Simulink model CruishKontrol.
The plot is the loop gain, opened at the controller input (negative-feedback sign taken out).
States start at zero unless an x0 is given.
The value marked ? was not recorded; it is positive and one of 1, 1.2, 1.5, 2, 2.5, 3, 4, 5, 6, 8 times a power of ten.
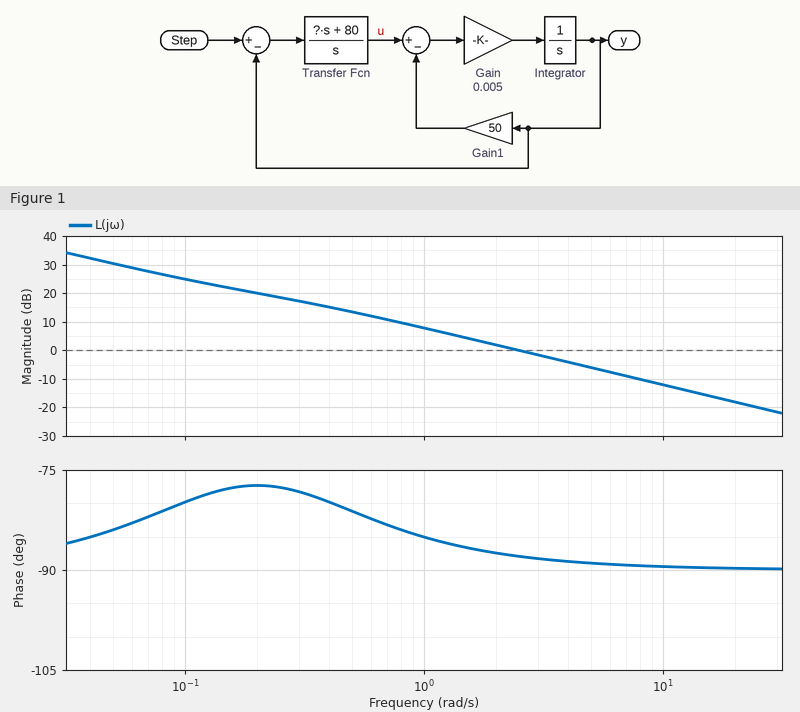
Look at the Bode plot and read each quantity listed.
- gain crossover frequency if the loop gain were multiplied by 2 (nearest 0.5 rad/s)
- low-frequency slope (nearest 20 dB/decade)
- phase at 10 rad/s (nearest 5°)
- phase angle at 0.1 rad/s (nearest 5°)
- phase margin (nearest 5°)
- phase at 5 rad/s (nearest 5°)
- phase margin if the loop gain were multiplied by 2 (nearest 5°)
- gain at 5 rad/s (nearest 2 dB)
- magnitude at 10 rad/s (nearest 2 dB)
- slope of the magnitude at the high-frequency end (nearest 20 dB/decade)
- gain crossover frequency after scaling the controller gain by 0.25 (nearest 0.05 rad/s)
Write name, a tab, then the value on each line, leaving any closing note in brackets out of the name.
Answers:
gain crossover frequency if the loop gain were multiplied by 2	5.0 rad/s
low-frequency slope	-20 dB/decade
phase at 10 rad/s	-90°
phase angle at 0.1 rad/s	-80°
phase margin	90°
phase at 5 rad/s	-90°
phase margin if the loop gain were multiplied by 2	90°
gain at 5 rad/s	-6 dB
magnitude at 10 rad/s	-12 dB
slope of the magnitude at the high-frequency end	-20 dB/decade
gain crossover frequency after scaling the controller gain by 0.25	0.60 rad/s
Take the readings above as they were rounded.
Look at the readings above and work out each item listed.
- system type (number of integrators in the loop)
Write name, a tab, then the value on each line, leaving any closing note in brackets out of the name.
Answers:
system type	1
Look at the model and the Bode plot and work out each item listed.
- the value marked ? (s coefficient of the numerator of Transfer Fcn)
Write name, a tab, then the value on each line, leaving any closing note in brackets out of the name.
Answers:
the value marked ?	500
